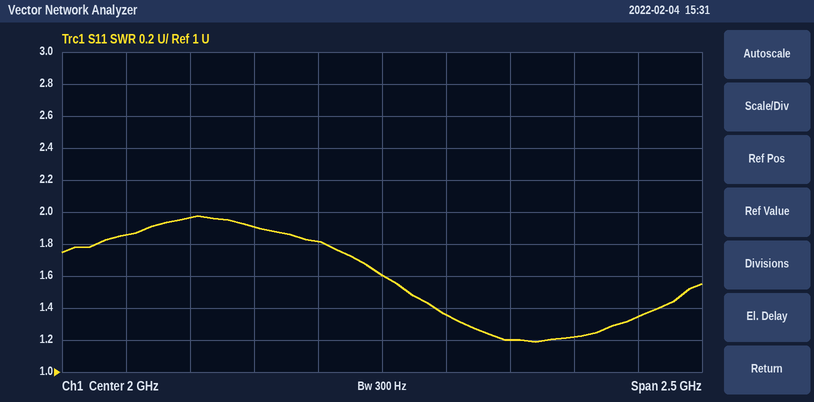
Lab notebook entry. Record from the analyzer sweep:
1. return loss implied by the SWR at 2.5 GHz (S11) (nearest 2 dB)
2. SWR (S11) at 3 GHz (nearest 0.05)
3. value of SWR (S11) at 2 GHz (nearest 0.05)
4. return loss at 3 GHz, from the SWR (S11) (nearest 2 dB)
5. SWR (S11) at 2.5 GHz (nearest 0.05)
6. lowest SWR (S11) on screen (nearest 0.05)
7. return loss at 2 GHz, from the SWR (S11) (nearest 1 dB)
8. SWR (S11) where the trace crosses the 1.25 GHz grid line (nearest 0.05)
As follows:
20 dB
1.35
1.60
16 dB
1.20
1.20
13 dB
1.95
